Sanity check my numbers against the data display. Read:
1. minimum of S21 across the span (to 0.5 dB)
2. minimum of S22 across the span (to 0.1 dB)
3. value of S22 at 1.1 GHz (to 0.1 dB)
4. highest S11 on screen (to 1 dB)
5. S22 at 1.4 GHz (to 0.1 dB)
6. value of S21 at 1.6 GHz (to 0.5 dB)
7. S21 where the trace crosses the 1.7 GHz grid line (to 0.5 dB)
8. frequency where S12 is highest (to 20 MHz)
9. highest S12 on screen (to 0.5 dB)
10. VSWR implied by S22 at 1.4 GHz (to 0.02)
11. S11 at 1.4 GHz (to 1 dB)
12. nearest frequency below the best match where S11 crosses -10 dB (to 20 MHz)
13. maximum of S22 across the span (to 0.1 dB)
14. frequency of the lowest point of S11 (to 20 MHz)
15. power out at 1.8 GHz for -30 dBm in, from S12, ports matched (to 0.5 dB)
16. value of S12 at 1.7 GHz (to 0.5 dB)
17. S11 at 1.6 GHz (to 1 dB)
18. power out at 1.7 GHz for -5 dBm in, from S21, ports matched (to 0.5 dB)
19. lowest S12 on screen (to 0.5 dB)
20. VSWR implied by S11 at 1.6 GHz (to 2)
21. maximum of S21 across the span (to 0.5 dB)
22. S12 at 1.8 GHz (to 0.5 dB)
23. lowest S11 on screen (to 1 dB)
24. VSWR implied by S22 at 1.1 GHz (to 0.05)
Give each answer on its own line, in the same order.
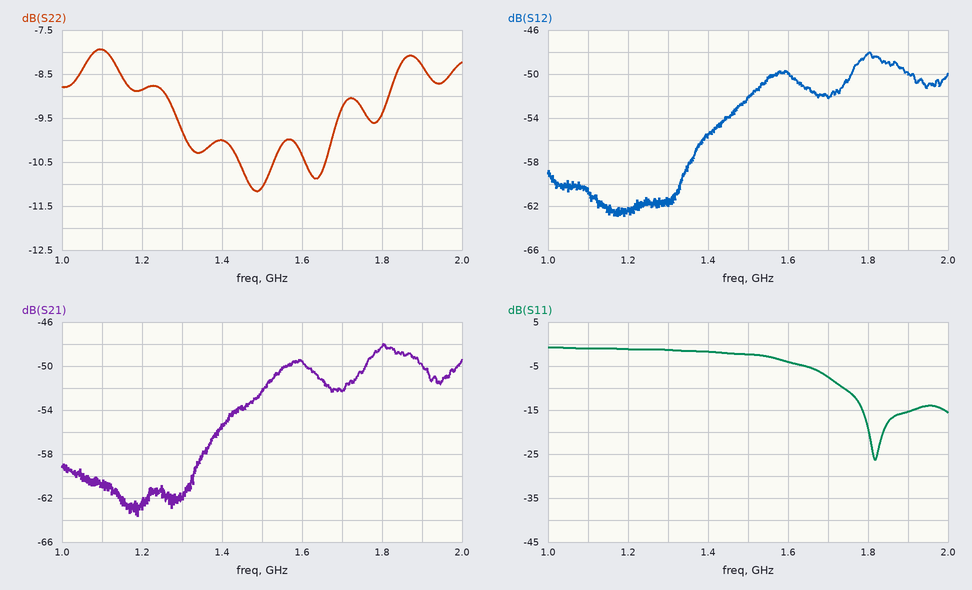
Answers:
-63.5 dB
-11.2 dB
-7.9 dB
-1 dB
-10.0 dB
-49.5 dB
-52.0 dB
1.80 GHz
-48.0 dB
1.92
-2 dB
1.74 GHz
-7.9 dB
1.82 GHz
-78.0 dBm
-52.0 dB
-4 dB
-57.0 dBm
-63.0 dB
4
-48.0 dB
-48.0 dB
-26 dB
2.35
